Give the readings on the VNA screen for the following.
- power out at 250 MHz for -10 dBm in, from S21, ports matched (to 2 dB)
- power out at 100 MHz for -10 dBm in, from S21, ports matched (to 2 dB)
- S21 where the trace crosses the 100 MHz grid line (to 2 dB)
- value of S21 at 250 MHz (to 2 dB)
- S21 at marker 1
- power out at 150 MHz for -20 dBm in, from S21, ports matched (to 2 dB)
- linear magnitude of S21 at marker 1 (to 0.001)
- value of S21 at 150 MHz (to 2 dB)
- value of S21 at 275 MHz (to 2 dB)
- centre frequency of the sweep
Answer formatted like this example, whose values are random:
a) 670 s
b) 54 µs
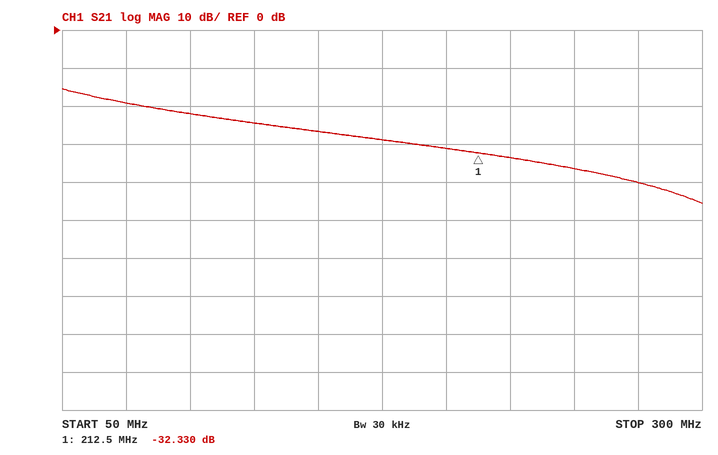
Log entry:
a) -46 dBm
b) -32 dBm
c) -22 dB
d) -36 dB
e) -32.330 dB
f) -46 dBm
g) 0.024
h) -26 dB
i) -40 dB
j) 175 MHz
